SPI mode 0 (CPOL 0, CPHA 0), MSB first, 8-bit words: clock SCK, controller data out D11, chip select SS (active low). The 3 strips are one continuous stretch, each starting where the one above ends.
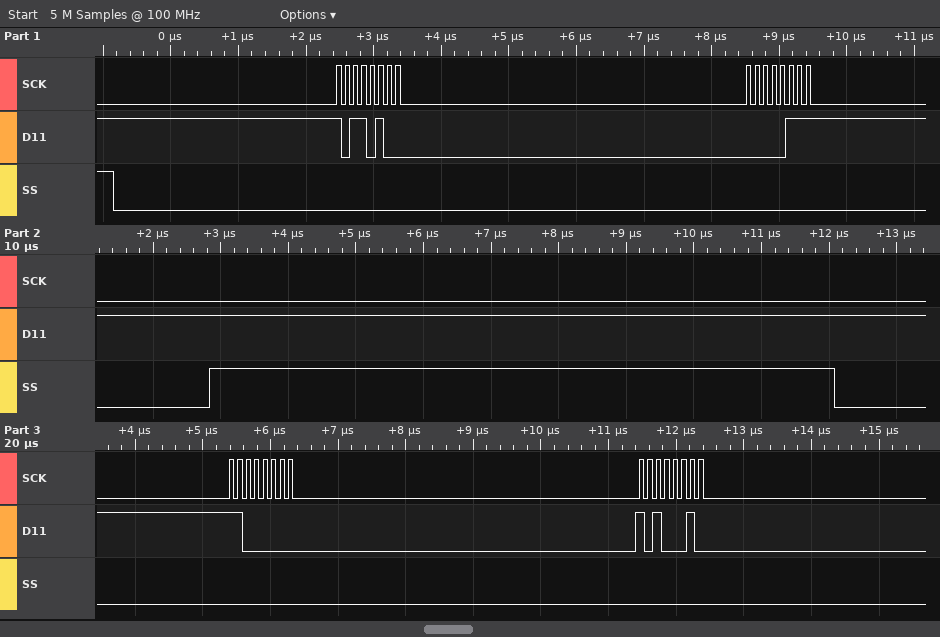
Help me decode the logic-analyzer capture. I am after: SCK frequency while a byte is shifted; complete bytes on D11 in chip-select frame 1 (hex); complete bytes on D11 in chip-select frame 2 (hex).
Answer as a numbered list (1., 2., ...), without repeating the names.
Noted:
1. 8 MHz
2. 0xB4 0x07
3. 0xC0 0xA2
